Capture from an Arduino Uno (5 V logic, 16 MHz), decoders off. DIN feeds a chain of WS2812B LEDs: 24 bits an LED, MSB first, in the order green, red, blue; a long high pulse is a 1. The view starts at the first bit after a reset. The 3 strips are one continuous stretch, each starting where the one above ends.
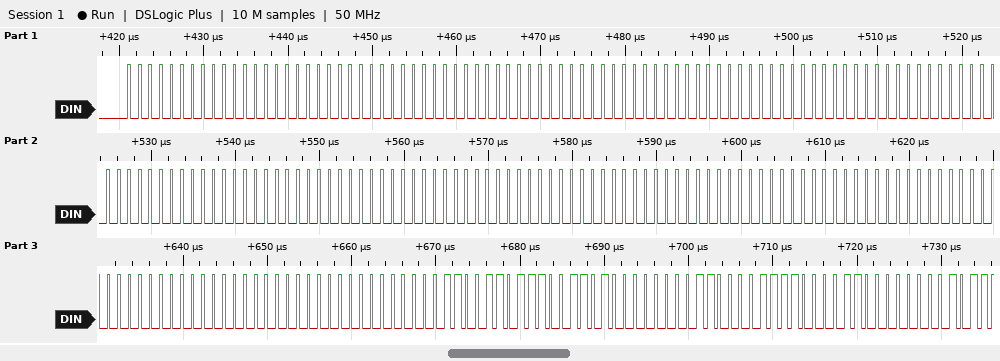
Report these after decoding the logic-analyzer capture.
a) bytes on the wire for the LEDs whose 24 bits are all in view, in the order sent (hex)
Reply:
00 00 00 00 00 00 00 00 00 00 00 00 00 00 00 00 00 00 00 00 00 00 00 00 00 CD CD 00 C3 C3
